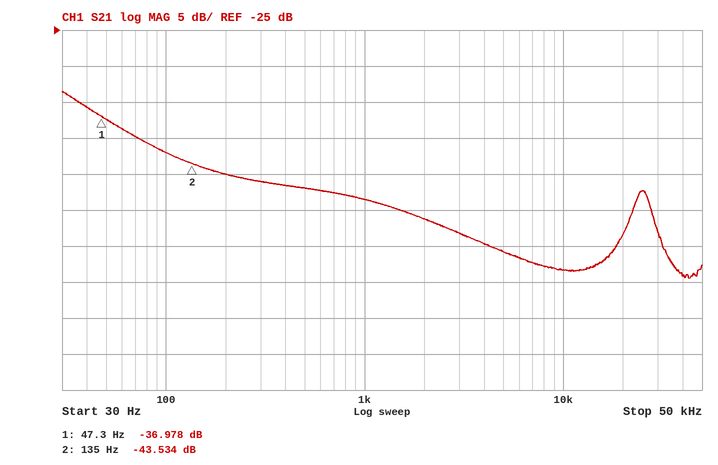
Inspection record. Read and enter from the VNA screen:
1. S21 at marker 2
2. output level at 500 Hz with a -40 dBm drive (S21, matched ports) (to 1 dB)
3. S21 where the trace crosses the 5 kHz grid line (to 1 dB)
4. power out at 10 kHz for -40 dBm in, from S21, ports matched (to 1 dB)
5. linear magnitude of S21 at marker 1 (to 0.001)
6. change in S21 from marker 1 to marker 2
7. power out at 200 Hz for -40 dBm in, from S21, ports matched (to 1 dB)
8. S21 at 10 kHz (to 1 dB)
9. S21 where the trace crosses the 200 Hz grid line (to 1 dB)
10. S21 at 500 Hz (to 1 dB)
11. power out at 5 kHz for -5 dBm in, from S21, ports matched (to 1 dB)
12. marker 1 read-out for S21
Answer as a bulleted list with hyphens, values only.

- -43.534 dB
- -87 dBm
- -56 dB
- -98 dBm
- 0.014
- -6.556 dB
- -85 dBm
- -58 dB
- -45 dB
- -47 dB
- -61 dBm
- -36.978 dB
